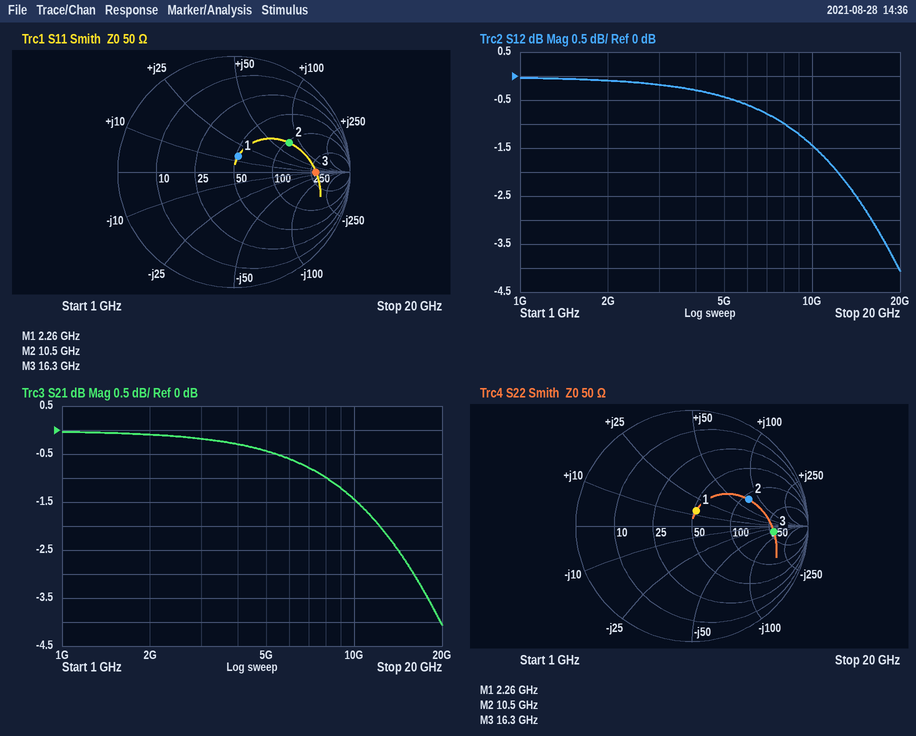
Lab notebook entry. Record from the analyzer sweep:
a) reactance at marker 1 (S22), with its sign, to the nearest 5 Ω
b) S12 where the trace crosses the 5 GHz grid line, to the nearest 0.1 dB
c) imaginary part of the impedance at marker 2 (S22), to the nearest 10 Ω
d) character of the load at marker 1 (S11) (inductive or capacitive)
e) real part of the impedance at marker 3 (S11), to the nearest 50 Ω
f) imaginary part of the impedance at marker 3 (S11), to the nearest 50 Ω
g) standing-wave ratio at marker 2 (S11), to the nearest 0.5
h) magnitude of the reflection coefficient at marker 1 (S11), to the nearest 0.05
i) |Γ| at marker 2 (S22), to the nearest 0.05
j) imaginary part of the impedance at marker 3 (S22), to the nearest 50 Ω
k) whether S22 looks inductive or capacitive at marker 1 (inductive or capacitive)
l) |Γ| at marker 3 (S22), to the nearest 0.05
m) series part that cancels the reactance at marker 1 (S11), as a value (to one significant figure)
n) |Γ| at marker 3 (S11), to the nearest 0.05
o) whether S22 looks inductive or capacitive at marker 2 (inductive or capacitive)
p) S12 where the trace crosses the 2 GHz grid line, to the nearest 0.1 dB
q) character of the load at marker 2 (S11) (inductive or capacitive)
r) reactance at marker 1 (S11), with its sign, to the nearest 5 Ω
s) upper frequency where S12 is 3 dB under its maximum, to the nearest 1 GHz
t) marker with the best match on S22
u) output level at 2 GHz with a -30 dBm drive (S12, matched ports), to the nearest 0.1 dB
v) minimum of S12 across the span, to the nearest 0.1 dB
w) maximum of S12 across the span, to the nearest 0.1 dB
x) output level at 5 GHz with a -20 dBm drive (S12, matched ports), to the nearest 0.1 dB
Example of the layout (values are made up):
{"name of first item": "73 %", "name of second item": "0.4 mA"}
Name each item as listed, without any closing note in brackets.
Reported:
{"reactance at marker 1 (S22), with its sign, to the nearest 5 Ω": "+15 Ω", "S12 where the trace crosses the 5 GHz grid line, to the nearest 0.1 dB": "-0.4 dB", "imaginary part of the impedance at marker 2 (S22), to the nearest 10 Ω": "+70 Ω", "character of the load at marker 1 (S11)": "inductive", "real part of the impedance at marker 3 (S11), to the nearest 50 Ω": "300 Ω", "imaginary part of the impedance at marker 3 (S11), to the nearest 50 Ω": "0 Ω", "standing-wave ratio at marker 2 (S11), to the nearest 0.5": "3.5", "magnitude of the reflection coefficient at marker 1 (S11), to the nearest 0.05": "0.15", "|Γ| at marker 2 (S22), to the nearest 0.05": "0.55", "imaginary part of the impedance at marker 3 (S22), to the nearest 50 Ω": "-50 Ω", "whether S22 looks inductive or capacitive at marker 1": "inductive", "|Γ| at marker 3 (S22), to the nearest 0.05": "0.70", "series part that cancels the reactance at marker 1 (S11), as a value": "5 pF", "|Γ| at marker 3 (S11), to the nearest 0.05": "0.70", "whether S22 looks inductive or capacitive at marker 2": "inductive", "S12 where the trace crosses the 2 GHz grid line, to the nearest 0.1 dB": "-0.1 dB", "character of the load at marker 2 (S11)": "inductive", "reactance at marker 1 (S11), with its sign, to the nearest 5 Ω": "+15 Ω", "upper frequency where S12 is 3 dB under its maximum, to the nearest 1 GHz": "16 GHz", "marker with the best match on S22": "marker 1", "output level at 2 GHz with a -30 dBm drive (S12, matched ports), to the nearest 0.1 dB": "-30.1 dBm", "minimum of S12 across the span, to the nearest 0.1 dB": "-4.1 dB", "maximum of S12 across the span, to the nearest 0.1 dB": "0.0 dB", "output level at 5 GHz with a -20 dBm drive (S12, matched ports), to the nearest 0.1 dB": "-20.4 dBm"}
